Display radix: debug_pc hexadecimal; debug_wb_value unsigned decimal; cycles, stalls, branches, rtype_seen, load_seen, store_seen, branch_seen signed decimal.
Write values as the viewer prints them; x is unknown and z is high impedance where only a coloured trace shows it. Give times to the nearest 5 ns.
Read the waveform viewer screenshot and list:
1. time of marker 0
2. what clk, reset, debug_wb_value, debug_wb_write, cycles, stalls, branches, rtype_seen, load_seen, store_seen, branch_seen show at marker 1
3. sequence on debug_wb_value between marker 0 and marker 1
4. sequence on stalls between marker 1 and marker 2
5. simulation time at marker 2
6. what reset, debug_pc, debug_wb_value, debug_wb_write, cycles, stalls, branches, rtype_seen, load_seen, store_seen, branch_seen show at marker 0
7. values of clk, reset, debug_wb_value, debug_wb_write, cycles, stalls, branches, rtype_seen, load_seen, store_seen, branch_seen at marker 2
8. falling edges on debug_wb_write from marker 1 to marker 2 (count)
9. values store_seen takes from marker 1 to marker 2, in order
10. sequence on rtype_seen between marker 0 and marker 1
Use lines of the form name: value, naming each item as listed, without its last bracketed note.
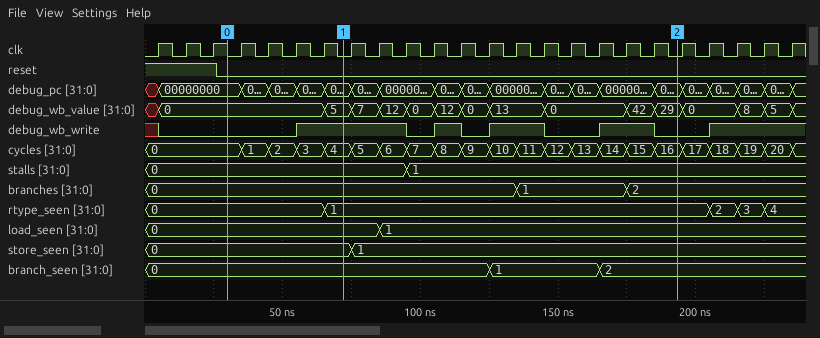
time of marker 0: 30 ns
what clk, reset, debug_wb_value, debug_wb_write, cycles, stalls, branches, rtype_seen, load_seen, store_seen, branch_seen show at marker 1: clk=0, reset=0, debug_wb_value=5, debug_wb_write=1, cycles=4, stalls=0, branches=0, rtype_seen=1, load_seen=0, store_seen=0, branch_seen=0
sequence on debug_wb_value between marker 0 and marker 1: 0, 5
sequence on stalls between marker 1 and marker 2: 0, 1
simulation time at marker 2: 195 ns
what reset, debug_pc, debug_wb_value, debug_wb_write, cycles, stalls, branches, rtype_seen, load_seen, store_seen, branch_seen show at marker 0: reset=0, debug_pc=00000000, debug_wb_value=0, debug_wb_write=0, cycles=0, stalls=0, branches=0, rtype_seen=0, load_seen=0, store_seen=0, branch_seen=0
values of clk, reset, debug_wb_value, debug_wb_write, cycles, stalls, branches, rtype_seen, load_seen, store_seen, branch_seen at marker 2: clk=0, reset=0, debug_wb_value=29, debug_wb_write=0, cycles=16, stalls=1, branches=2, rtype_seen=1, load_seen=1, store_seen=1, branch_seen=2
falling edges on debug_wb_write from marker 1 to marker 2: 4
values store_seen takes from marker 1 to marker 2, in order: 0, 1
sequence on rtype_seen between marker 0 and marker 1: 0, 1
